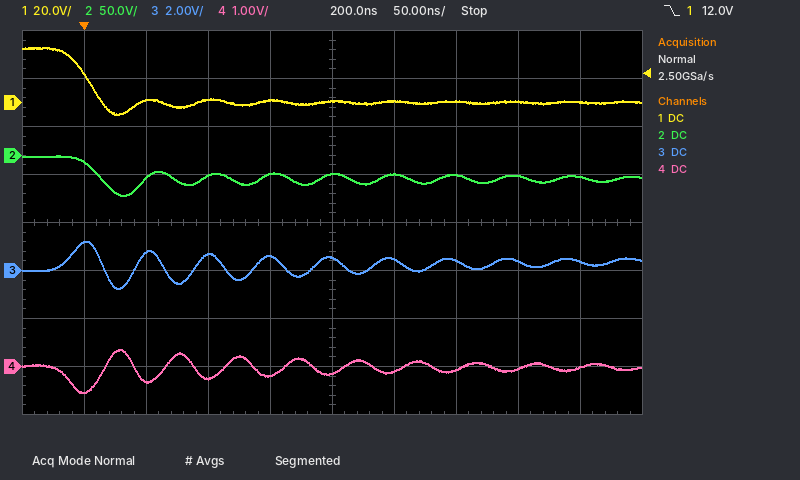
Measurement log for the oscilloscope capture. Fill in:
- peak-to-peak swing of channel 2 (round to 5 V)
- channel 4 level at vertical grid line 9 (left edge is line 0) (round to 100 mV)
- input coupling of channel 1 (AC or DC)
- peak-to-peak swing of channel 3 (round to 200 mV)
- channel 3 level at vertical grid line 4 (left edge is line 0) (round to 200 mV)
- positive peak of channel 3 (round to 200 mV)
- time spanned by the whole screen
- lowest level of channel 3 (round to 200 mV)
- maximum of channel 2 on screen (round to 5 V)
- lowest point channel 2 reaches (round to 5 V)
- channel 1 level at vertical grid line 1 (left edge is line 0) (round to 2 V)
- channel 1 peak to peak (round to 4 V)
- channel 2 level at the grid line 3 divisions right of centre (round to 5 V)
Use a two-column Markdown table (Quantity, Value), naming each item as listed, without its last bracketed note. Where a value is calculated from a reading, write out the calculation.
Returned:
| Quantity | Value |
|---|---|
| peak-to-peak swing of channel 2 | 0 V − (-40 V) = 40 V |
| channel 4 level at vertical grid line 9 (left edge is line 0) | 0.0 V |
| input coupling of channel 1 | DC |
| peak-to-peak swing of channel 3 | 1.2 V − (-800 mV) = 2.0 V |
| channel 3 level at vertical grid line 4 (left edge is line 0) | 600 mV |
| positive peak of channel 3 | 1.2 V |
| time spanned by the whole screen | 500 ns |
| lowest level of channel 3 | -800 mV |
| maximum of channel 2 on screen | 0 V |
| lowest point channel 2 reaches | -40 V |
| channel 1 level at vertical grid line 1 (left edge is line 0) | 12 V |
| channel 1 peak to peak | 28 V |
| channel 2 level at the grid line 3 divisions right of centre | -20 V |
